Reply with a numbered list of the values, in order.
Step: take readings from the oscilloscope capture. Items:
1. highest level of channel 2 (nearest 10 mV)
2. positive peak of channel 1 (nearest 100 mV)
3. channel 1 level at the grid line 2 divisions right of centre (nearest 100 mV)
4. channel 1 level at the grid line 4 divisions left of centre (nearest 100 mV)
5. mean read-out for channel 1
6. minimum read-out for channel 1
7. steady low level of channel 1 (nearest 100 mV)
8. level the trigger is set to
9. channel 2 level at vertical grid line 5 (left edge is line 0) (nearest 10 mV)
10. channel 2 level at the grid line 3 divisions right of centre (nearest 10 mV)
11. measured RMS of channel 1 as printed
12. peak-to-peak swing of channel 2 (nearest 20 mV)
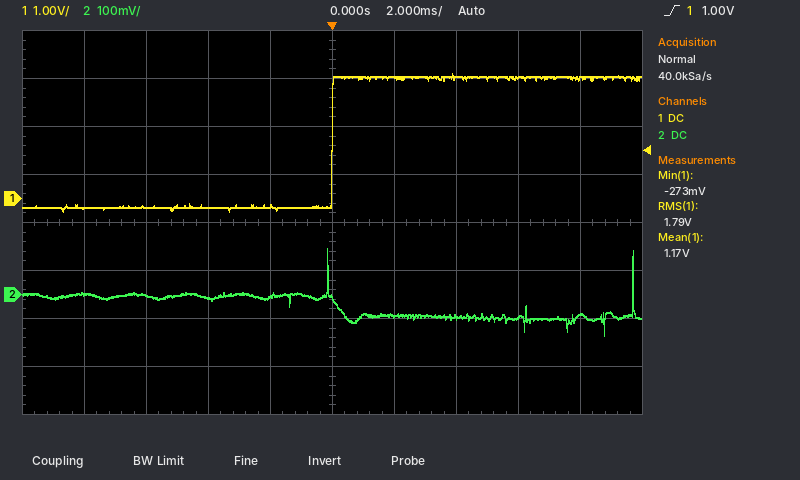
1. 100 mV
2. 2.6 V
3. 2.5 V
4. -200 mV
5. 1.17 V
6. -273 mV
7. -200 mV
8. 1.00 V
9. -10 mV
10. -50 mV
11. 1.79 V
12. 180 mV
